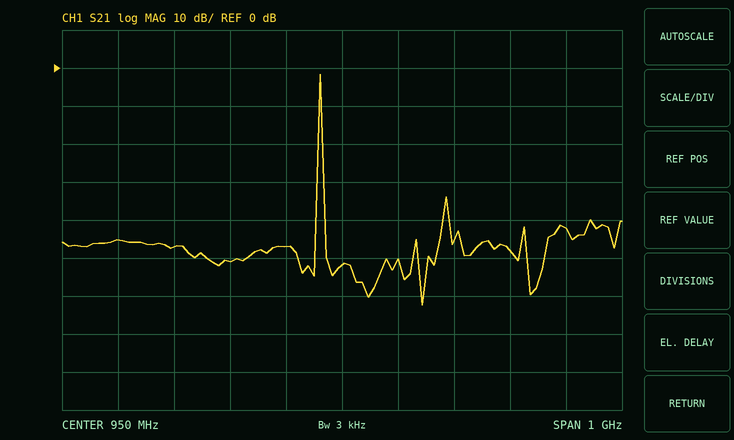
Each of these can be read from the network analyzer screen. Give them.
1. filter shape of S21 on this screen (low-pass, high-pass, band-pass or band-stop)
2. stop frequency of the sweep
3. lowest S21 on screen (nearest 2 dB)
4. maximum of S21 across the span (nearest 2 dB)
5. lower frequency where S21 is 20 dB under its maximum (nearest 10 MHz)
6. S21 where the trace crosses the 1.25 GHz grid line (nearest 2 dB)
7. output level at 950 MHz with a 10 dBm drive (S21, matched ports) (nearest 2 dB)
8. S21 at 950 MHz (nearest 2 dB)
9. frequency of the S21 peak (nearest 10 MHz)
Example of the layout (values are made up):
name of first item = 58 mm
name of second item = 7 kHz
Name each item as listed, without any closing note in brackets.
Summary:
filter shape of S21 on this screen = band-pass
stop frequency of the sweep = 1.45 GHz
lowest S21 on screen = -62 dB
maximum of S21 across the span = -2 dB
lower frequency where S21 is 20 dB under its maximum = 910 MHz
S21 where the trace crosses the 1.25 GHz grid line = -48 dB
output level at 950 MHz with a 10 dBm drive (S21, matched ports) = -42 dBm
S21 at 950 MHz = -52 dB
frequency of the S21 peak = 910 MHz
